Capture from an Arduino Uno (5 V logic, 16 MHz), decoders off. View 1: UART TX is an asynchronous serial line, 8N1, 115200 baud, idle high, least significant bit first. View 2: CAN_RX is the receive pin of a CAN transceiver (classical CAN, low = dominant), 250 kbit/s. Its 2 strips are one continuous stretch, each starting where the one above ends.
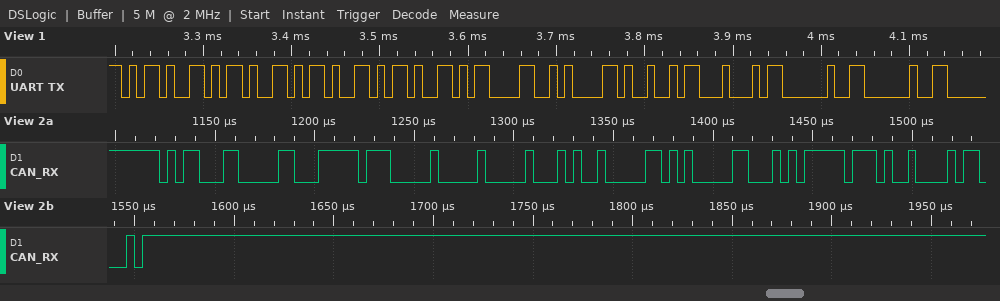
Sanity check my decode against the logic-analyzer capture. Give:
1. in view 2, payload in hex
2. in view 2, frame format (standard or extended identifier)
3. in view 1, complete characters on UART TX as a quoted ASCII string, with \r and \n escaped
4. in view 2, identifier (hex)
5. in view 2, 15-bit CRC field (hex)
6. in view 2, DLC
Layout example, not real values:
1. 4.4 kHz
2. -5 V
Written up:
1. FF 00 00 29 05 41 15 FE
2. standard
3. "----\r\nID  "
4. 0x58C
5. 0x4858
6. 8
